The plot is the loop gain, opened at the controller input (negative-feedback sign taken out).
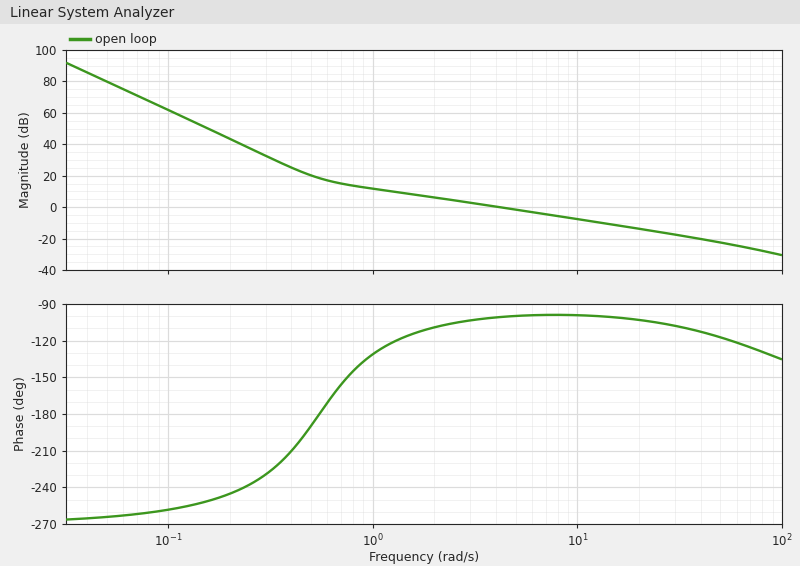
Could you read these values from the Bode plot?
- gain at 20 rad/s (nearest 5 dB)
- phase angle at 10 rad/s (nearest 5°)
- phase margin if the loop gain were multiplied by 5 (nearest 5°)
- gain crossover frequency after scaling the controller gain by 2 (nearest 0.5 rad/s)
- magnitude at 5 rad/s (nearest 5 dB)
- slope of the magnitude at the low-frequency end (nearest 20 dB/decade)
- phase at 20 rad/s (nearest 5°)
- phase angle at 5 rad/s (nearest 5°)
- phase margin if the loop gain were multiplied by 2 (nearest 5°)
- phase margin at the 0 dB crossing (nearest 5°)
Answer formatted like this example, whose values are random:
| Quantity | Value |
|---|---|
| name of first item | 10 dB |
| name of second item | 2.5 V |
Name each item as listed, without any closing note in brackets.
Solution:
| Quantity | Value |
|---|---|
| gain at 20 rad/s | -15 dB |
| phase angle at 10 rad/s | -100° |
| phase margin if the loop gain were multiplied by 5 | 75° |
| gain crossover frequency after scaling the controller gain by 2 | 8.5 rad/s |
| magnitude at 5 rad/s | 0 dB |
| slope of the magnitude at the low-frequency end | -60 dB/decade |
| phase at 20 rad/s | -105° |
| phase angle at 5 rad/s | -100° |
| phase margin if the loop gain were multiplied by 2 | 80° |
| phase margin at the 0 dB crossing | 80° |
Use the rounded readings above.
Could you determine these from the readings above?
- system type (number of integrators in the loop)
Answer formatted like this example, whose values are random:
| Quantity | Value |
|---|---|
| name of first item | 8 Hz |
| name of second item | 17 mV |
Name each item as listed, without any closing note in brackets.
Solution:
| Quantity | Value |
|---|---|
| system type | 3 |
